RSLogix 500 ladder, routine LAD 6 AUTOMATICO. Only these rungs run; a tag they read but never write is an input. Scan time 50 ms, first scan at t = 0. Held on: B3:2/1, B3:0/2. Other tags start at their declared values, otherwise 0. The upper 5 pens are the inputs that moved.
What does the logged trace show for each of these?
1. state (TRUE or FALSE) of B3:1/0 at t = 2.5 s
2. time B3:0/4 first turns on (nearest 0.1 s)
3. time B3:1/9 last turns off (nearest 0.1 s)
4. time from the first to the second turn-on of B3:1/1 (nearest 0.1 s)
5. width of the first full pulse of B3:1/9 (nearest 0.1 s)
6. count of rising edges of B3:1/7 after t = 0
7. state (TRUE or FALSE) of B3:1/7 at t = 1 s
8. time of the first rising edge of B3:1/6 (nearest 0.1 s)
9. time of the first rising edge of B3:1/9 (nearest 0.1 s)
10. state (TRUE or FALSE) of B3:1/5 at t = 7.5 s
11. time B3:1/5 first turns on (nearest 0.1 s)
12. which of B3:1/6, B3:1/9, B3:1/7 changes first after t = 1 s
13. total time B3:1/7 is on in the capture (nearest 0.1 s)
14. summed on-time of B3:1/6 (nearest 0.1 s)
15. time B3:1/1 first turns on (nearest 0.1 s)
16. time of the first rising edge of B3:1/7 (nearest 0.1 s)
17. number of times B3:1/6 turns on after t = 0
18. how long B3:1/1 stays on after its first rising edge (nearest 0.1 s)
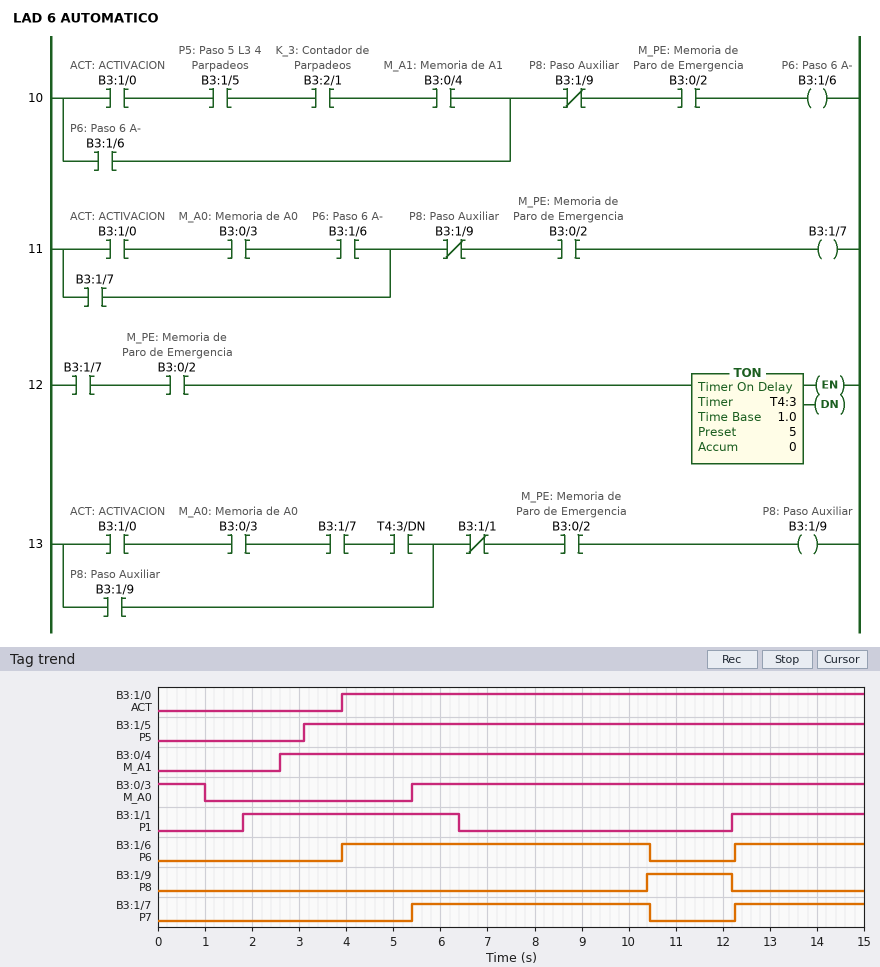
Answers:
FALSE
2.6 s
12.2 s
10.4 s
1.8 s
2
FALSE
3.9 s
10.4 s
TRUE
3.1 s
B3:1/6
7.8 s
9.3 s
1.8 s
5.4 s
2
4.6 s
